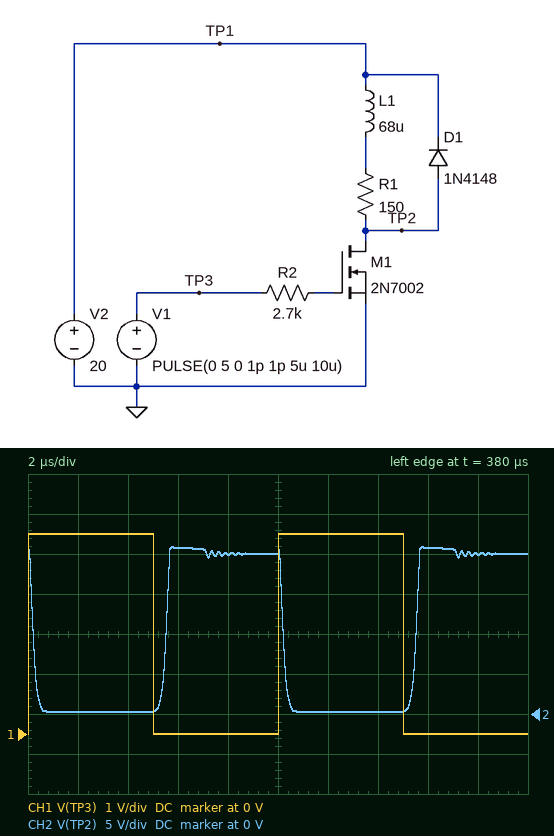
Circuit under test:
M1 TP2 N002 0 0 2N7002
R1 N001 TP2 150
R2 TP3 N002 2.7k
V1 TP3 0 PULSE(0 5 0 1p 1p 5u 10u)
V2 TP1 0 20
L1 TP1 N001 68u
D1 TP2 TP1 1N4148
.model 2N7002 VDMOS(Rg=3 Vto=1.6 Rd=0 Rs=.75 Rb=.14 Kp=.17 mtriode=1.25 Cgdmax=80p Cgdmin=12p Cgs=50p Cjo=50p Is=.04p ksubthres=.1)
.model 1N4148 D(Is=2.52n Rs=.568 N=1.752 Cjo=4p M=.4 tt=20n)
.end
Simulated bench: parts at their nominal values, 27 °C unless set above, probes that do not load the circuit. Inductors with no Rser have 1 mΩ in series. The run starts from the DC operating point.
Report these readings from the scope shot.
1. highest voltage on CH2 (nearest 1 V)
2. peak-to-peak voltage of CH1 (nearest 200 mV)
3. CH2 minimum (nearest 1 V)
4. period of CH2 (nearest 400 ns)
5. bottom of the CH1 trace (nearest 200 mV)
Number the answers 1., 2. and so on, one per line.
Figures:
1. 21 V
2. 5.0 V
3. 0 V
4. 10.0 µs
5. 0 V
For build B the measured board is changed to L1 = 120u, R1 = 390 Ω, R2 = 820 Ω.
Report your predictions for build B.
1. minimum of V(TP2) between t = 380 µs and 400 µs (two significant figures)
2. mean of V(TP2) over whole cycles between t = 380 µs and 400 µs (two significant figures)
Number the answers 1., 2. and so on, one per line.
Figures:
1. 69 mV
2. 9.9 V
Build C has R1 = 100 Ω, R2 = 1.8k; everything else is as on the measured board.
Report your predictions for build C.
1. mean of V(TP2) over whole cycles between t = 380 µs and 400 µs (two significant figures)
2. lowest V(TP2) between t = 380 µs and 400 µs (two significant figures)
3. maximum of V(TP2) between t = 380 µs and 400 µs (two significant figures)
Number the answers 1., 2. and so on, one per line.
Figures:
1. 10 V
2. 270 mV
3. 21 V
